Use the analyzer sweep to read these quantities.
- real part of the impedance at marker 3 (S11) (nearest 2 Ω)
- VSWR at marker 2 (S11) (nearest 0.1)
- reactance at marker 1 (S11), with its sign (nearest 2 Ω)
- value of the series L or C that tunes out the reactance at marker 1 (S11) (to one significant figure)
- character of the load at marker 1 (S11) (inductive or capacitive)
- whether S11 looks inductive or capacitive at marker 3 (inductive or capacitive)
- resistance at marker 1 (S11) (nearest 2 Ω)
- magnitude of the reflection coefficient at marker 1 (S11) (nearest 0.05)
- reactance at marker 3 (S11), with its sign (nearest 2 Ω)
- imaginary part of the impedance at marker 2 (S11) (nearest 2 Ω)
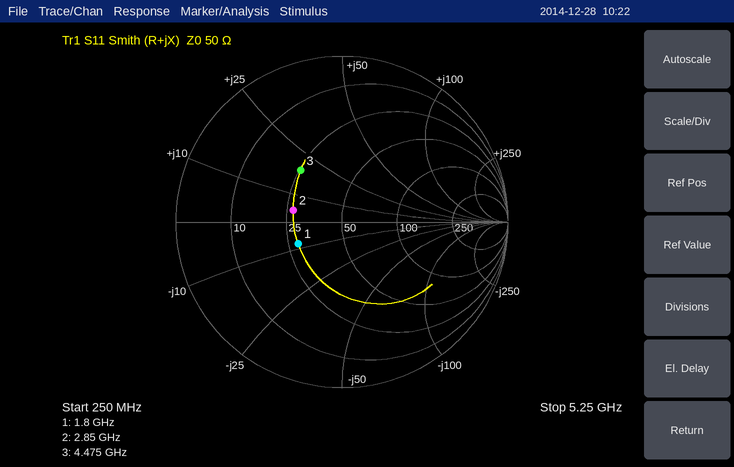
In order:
26 Ω
1.9
-8 Ω
700 pH
capacitive
inductive
28 Ω
0.30
+18 Ω
+4 Ω
